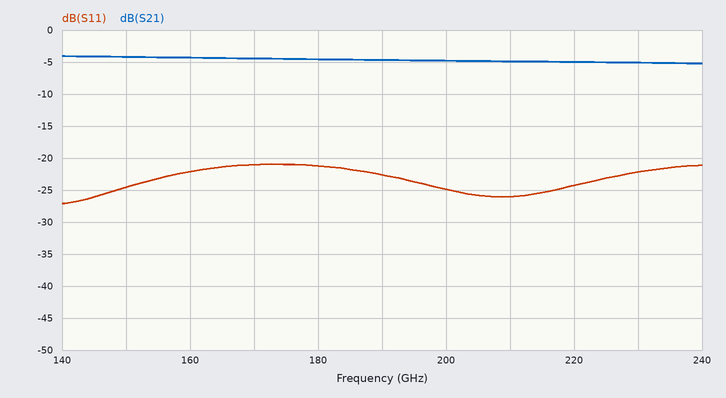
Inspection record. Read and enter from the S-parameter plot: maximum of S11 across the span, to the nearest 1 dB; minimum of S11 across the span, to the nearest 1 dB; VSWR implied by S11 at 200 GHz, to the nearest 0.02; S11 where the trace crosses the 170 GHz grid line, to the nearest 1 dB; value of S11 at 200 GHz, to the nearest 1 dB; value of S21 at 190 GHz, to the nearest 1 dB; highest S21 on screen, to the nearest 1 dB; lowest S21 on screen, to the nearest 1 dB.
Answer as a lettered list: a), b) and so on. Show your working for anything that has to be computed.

a) -21 dB
b) -27 dB
c) |Γ| = 10^(-25/20) = 0.0562; VSWR = (1 + 0.0562)/(1 − 0.0562) ≈ 1.12
d) -21 dB
e) -25 dB
f) -5 dB
g) -4 dB
h) -5 dB
